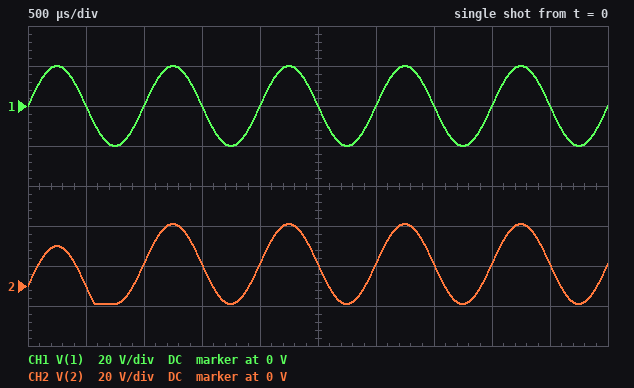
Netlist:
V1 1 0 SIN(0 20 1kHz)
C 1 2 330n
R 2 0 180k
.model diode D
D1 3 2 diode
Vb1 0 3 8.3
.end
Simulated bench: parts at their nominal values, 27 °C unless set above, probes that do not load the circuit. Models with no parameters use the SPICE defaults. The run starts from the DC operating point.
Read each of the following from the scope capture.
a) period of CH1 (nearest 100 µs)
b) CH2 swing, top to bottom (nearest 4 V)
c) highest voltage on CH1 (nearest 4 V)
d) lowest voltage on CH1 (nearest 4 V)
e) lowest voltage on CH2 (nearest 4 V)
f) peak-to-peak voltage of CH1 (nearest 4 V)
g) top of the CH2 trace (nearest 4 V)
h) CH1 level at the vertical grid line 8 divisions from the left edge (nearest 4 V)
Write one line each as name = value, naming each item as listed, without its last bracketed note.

period of CH1 = 1.0 ms
CH2 swing, top to bottom = 40 V
highest voltage on CH1 = 20 V
lowest voltage on CH1 = -20 V
lowest voltage on CH2 = -8 V
peak-to-peak voltage of CH1 = 40 V
top of the CH2 trace = 32 V
CH1 level at the vertical grid line 8 divisions from the left edge = 0 V
